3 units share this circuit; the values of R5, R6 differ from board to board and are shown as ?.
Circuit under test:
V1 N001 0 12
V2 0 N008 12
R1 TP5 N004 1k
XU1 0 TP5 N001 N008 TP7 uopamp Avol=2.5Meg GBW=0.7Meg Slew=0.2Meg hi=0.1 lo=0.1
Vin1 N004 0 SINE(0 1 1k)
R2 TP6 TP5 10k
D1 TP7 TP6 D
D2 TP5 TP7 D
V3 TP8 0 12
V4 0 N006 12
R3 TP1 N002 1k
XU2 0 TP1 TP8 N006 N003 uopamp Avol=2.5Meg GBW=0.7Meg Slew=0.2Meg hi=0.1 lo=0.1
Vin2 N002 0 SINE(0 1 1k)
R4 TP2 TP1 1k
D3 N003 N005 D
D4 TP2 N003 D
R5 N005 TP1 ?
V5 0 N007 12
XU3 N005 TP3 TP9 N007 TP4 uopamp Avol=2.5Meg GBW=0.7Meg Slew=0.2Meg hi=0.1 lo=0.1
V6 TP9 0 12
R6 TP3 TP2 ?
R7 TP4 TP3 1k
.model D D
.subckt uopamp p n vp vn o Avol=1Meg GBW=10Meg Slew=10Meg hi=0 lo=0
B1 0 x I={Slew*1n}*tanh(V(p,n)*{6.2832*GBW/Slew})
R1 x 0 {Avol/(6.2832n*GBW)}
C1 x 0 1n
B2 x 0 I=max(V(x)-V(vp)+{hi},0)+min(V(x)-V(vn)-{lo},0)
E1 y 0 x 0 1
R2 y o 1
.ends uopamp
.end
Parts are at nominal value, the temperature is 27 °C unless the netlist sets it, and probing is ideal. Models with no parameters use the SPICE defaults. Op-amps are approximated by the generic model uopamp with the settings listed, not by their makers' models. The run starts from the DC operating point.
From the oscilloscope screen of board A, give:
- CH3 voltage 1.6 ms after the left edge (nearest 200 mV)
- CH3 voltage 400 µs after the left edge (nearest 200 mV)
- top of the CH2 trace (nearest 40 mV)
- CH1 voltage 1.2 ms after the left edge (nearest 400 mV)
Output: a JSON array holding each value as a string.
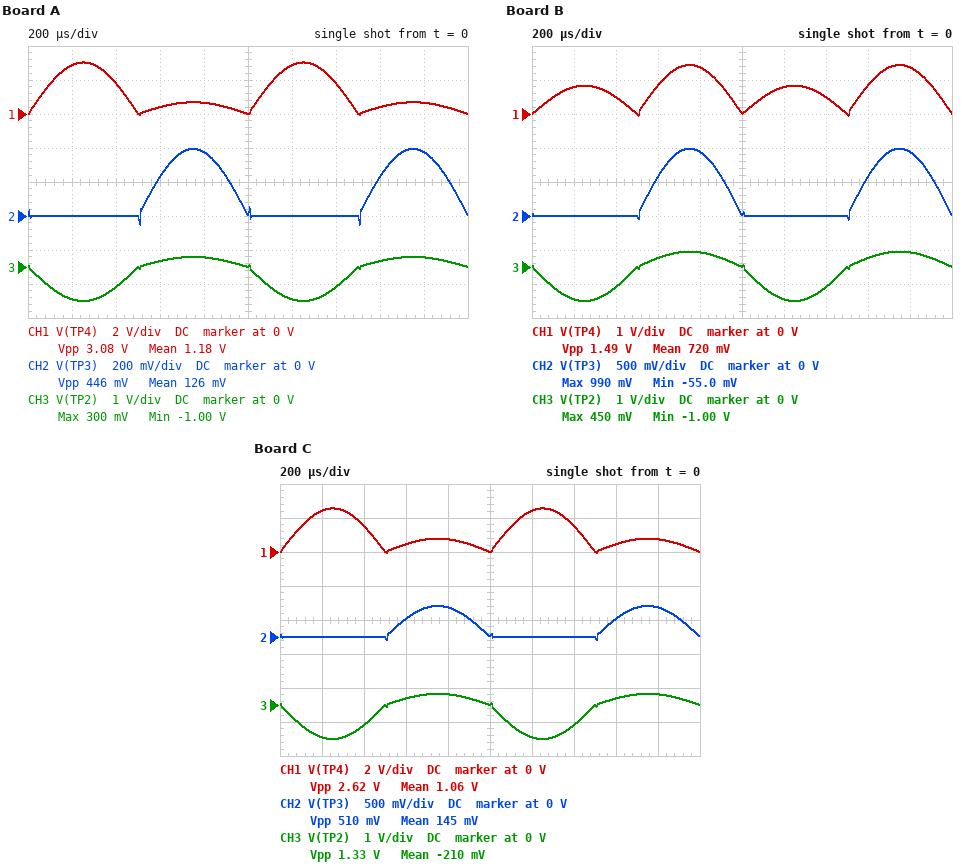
["200 mV", "-600 mV", "400 mV", "2.8 V"]
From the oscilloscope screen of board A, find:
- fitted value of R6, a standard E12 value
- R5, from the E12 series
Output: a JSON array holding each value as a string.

["330 Ω", "560 Ω"]
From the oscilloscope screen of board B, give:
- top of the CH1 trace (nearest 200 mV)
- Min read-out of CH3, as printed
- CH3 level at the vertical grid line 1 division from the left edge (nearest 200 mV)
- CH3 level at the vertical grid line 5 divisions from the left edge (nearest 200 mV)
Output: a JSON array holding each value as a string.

["1.4 V", "-1.00 V", "-1.0 V", "0 V"]
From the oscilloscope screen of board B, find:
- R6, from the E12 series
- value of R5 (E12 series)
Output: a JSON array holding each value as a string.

["1.2 kΩ", "1.8 kΩ"]
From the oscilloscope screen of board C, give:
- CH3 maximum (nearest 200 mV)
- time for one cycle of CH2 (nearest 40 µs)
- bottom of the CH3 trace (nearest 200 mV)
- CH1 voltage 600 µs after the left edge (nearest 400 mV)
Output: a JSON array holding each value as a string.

["400 mV", "1.00 ms", "-1.0 V", "400 mV"]
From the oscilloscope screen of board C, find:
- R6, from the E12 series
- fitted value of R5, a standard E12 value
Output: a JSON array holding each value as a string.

["390 Ω", "680 Ω"]
